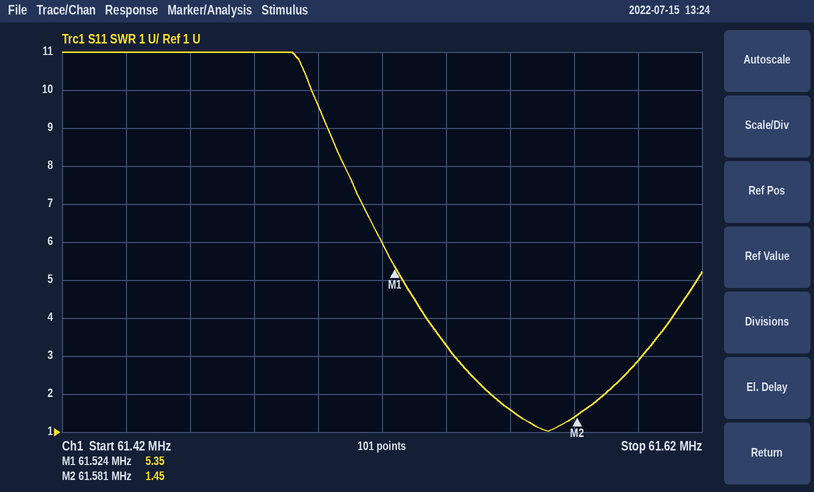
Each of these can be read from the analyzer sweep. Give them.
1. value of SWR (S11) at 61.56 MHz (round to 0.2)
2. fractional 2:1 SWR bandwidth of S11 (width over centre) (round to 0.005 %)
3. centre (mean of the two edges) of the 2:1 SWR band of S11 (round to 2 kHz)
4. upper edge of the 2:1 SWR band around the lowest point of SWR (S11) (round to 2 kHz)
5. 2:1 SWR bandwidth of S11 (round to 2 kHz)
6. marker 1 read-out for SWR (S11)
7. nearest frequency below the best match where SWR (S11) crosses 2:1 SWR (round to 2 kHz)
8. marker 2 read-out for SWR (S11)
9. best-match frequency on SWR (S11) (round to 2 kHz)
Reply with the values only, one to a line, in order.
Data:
1.6
0.060 %
61.572 MHz
61.590 MHz
36 kHz
5.35
61.554 MHz
1.45
61.572 MHz
